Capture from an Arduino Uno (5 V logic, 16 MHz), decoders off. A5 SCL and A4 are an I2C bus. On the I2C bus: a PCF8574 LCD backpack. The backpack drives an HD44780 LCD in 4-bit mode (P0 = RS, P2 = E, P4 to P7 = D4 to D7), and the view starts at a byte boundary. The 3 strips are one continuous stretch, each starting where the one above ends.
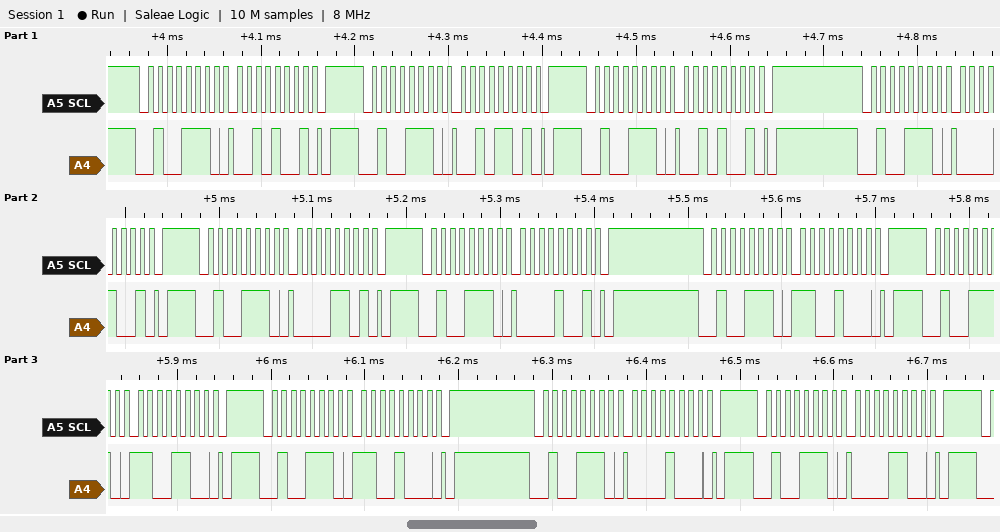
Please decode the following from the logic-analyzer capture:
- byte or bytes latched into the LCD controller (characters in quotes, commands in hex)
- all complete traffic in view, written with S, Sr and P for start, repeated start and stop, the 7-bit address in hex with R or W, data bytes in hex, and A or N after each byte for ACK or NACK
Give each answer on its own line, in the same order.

' '
S 27W A 29 A P S 27W A 2D A P S 27W A 29 A P S 27W A 09 A P S 27W A 0D A P S 27W A 09 A P S 27W A C8 A P S 27W A CC A P S 27W A C8 A P S 27W A 08 A P S 27W A 0C A P
